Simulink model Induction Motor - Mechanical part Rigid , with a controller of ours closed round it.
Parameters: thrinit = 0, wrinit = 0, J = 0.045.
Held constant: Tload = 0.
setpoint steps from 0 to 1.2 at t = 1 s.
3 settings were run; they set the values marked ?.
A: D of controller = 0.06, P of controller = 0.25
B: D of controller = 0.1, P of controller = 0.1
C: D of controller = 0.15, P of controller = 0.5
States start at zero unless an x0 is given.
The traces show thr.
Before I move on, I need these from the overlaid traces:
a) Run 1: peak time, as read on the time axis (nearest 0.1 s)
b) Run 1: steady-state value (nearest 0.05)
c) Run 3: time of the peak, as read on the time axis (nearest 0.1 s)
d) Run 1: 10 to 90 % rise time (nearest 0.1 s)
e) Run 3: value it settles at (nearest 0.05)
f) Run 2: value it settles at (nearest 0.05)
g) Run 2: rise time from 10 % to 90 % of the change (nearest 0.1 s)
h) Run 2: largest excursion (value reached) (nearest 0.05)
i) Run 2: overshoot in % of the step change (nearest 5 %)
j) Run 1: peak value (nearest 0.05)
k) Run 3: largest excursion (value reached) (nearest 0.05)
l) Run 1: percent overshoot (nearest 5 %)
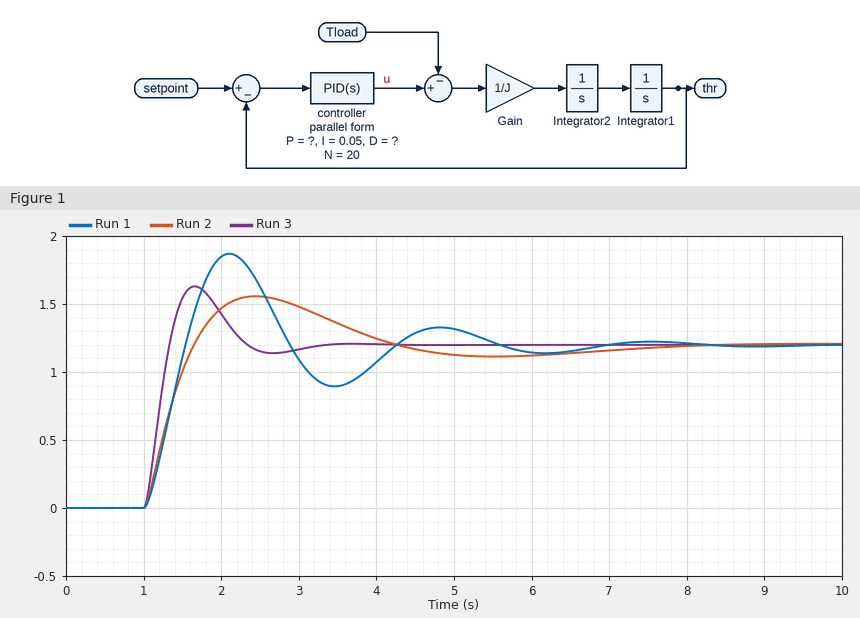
2.1 s
1.20
1.7 s
0.4 s
1.20
1.20
0.5 s
1.55
30 %
1.85
1.65
55 %
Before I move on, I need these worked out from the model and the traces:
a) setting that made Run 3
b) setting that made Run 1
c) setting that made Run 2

C
A
B
